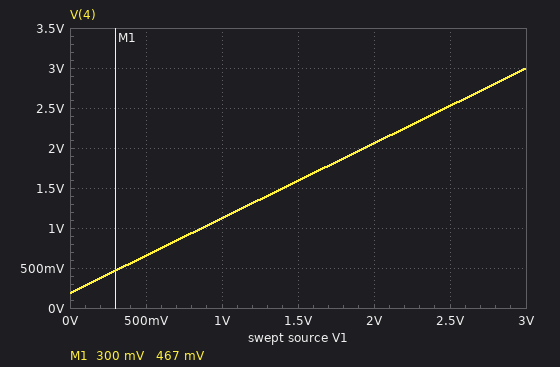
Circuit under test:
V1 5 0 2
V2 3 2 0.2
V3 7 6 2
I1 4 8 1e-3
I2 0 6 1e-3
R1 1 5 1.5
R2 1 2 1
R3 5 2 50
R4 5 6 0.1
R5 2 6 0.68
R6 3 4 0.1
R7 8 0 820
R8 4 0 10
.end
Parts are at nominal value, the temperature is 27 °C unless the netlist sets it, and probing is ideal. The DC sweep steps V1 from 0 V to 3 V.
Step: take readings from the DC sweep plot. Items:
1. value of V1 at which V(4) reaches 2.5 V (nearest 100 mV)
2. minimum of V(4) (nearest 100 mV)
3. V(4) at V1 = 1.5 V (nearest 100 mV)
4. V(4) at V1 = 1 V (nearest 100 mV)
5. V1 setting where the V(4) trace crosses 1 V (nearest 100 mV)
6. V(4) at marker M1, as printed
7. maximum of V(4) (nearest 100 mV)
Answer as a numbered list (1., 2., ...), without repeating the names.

1. 2.5 V
2. 200 mV
3. 1.6 V
4. 1.1 V
5. 900 mV
6. 467 mV
7. 3.0 V
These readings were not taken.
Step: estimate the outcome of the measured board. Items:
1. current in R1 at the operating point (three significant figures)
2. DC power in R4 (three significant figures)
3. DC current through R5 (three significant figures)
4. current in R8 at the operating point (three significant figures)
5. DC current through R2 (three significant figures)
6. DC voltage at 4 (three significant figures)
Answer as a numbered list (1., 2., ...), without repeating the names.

1. 48.6 mA
2. 2.40 mW
3. 156 mA
4. 206 mA
5. 48.6 mA
6. 2.06 V
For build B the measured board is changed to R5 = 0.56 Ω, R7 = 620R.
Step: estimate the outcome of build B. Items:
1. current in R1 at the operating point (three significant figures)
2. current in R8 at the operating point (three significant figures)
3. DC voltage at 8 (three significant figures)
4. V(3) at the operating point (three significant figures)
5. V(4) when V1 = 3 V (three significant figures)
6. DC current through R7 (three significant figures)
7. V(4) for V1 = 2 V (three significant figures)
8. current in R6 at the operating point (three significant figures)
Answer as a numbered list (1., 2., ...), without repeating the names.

1. 43.0 mA
2. 207 mA
3. 620 mV
4. 2.09 V
5. 3.01 V
6. 1.00 mA
7. 2.07 V
8. 208 mA
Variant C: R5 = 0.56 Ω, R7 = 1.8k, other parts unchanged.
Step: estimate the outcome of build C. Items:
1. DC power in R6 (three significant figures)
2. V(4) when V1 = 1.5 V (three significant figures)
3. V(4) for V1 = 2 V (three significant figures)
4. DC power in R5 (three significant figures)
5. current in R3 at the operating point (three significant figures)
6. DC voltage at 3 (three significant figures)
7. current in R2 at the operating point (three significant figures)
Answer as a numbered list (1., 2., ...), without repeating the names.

1. 4.33 mW
2. 1.60 V
3. 2.07 V
4. 14.9 mW
5. 2.15 mA
6. 2.09 V
7. 43.0 mA
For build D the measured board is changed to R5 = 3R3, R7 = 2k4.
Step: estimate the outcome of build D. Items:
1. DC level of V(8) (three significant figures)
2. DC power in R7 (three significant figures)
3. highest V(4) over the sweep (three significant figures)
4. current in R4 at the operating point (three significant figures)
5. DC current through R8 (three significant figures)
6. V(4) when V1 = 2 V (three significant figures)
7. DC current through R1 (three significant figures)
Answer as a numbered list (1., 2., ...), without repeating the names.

1. 2.40 V
2. 2.40 mW
3. 2.78 V
4. 78.2 mA
5. 191 mA
6. 1.91 V
7. 108 mA
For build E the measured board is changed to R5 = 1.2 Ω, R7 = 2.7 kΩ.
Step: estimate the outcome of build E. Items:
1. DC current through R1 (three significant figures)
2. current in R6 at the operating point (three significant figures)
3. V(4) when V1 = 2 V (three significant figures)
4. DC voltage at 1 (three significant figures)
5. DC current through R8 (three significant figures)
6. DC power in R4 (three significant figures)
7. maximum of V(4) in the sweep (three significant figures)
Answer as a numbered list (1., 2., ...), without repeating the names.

1. 67.9 mA
2. 202 mA
3. 2.01 V
4. 1.90 V
5. 201 mA
6. 1.68 mW
7. 2.92 V
